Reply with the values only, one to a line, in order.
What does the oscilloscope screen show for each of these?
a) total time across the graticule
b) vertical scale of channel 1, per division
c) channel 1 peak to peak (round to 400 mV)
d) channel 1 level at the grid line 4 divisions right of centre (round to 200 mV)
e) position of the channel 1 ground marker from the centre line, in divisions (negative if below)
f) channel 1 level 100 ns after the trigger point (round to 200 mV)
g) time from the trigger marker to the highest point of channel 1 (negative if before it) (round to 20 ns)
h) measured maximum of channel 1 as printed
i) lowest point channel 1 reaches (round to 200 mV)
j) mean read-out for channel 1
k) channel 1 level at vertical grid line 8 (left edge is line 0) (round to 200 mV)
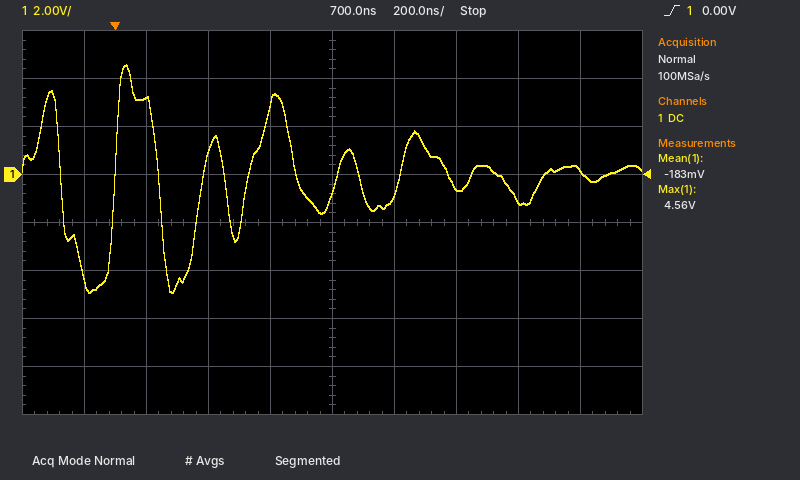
2 µs
2 V
9.6 V
200 mV
+1.0 div
3.2 V
+40 ns
4.56 V
-5.0 V
-183 mV
-1.0 V
